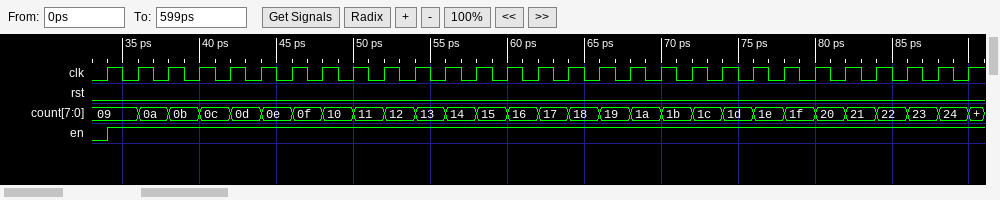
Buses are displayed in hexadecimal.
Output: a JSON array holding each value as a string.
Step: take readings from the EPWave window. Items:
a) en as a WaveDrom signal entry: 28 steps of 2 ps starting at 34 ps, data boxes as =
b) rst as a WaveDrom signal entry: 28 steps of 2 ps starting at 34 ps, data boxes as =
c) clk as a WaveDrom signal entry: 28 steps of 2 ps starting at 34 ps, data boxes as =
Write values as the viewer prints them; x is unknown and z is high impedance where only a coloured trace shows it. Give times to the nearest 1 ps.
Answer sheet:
["{name: 'en', wave: '1...........................'}", "{name: 'rst', wave: '0...........................'}", "{name: 'clk', wave: 'p...........................'}"]
